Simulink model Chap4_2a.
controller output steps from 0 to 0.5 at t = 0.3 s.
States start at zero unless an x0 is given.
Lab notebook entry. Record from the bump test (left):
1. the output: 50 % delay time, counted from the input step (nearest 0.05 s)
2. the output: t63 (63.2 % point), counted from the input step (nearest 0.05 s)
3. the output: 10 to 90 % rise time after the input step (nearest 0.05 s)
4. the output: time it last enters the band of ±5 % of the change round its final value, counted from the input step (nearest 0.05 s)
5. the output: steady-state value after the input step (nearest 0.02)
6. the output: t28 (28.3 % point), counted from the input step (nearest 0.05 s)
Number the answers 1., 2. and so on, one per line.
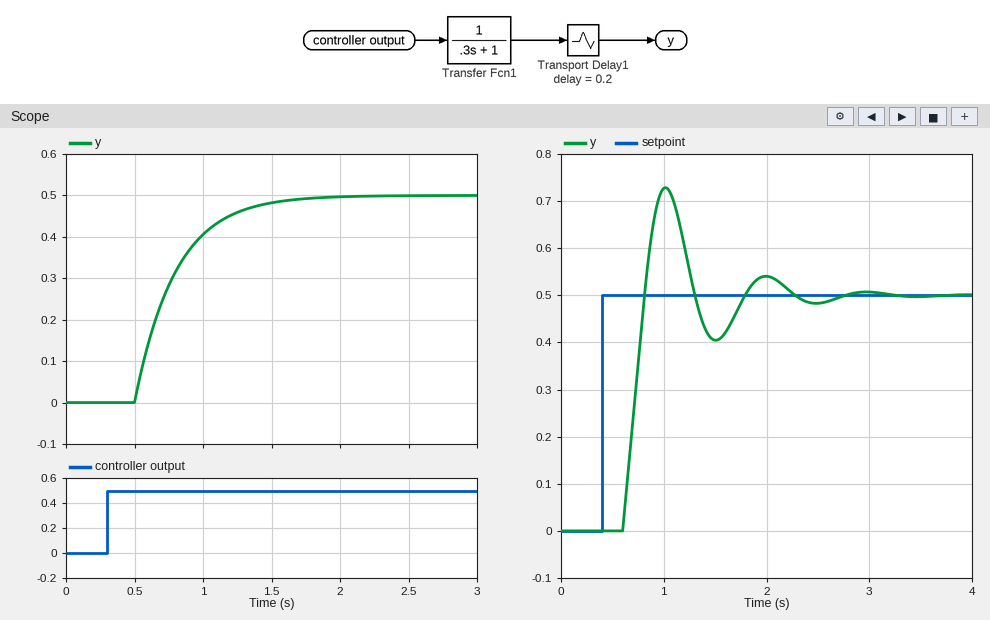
1. 0.40 s
2. 0.50 s
3. 0.65 s
4. 1.10 s
5. 0.50
6. 0.30 s
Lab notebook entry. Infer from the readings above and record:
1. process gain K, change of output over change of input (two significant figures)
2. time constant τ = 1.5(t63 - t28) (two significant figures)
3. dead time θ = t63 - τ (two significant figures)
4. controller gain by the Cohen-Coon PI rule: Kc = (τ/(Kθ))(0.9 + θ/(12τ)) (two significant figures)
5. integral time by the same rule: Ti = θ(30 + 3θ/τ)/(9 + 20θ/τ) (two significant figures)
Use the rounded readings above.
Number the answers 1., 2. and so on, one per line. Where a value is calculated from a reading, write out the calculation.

1. (0.5 - 0) / 0.5 = 1.0
2. 1.5 × (0.5 - 0.3) = 0.30 s
3. 0.5 - 0.3 = 0.20 s
4. 0.3 / (1 × 0.2) × (0.9 + 0.2 / (12 × 0.3)) = 1.4
5. 0.2 × (30 + 3 × 0.2 / 0.3) / (9 + 20 × 0.2 / 0.3) = 0.29 s
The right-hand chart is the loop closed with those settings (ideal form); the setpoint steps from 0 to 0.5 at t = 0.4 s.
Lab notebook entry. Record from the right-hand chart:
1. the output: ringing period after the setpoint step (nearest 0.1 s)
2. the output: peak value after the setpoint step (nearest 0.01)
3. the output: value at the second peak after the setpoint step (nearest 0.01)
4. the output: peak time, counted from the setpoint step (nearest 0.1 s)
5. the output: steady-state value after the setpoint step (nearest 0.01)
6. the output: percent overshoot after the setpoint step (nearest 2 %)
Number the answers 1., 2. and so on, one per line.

1. 1.0 s
2. 0.73
3. 0.54
4. 0.6 s
5. 0.50
6. 46 %
